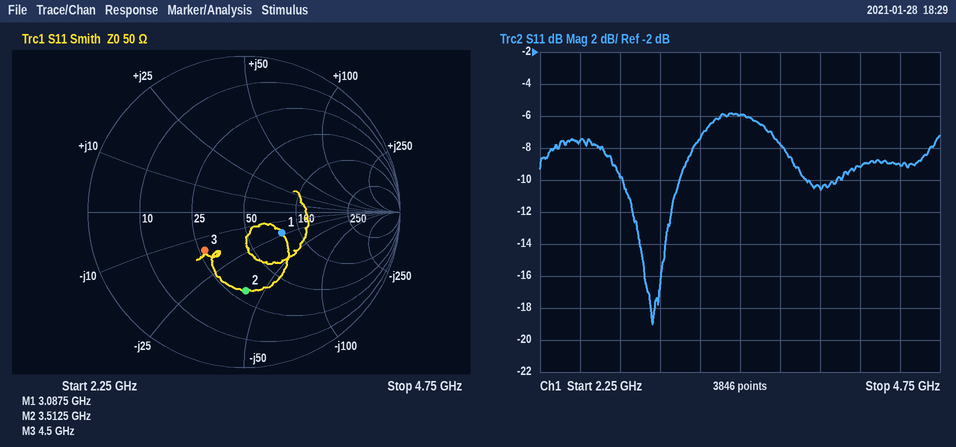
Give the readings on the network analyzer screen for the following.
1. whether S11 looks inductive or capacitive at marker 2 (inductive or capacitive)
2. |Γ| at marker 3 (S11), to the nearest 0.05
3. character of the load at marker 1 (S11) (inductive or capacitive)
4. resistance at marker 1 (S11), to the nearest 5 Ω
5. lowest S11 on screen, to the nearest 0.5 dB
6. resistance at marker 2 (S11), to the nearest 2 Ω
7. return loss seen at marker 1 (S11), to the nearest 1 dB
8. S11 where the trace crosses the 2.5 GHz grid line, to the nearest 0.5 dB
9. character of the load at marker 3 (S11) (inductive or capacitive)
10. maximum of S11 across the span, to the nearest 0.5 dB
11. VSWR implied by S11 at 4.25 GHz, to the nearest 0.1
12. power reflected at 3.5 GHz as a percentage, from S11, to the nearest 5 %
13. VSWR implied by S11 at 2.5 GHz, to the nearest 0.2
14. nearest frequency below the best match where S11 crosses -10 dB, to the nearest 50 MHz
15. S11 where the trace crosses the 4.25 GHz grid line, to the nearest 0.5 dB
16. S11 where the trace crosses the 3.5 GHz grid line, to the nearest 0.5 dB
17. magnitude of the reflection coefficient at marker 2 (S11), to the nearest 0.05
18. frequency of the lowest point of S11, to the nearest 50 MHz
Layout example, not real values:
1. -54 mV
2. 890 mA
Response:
1. capacitive
2. 0.35
3. capacitive
4. 80 Ω
5. -19.0 dB
6. 30 Ω
7. 11 dB
8. -7.5 dB
9. capacitive
10. -6.0 dB
11. 2.1
12. 25 %
13. 2.4
14. 2.75 GHz
15. -9.0 dB
16. -6.0 dB
17. 0.50
18. 2.95 GHz
